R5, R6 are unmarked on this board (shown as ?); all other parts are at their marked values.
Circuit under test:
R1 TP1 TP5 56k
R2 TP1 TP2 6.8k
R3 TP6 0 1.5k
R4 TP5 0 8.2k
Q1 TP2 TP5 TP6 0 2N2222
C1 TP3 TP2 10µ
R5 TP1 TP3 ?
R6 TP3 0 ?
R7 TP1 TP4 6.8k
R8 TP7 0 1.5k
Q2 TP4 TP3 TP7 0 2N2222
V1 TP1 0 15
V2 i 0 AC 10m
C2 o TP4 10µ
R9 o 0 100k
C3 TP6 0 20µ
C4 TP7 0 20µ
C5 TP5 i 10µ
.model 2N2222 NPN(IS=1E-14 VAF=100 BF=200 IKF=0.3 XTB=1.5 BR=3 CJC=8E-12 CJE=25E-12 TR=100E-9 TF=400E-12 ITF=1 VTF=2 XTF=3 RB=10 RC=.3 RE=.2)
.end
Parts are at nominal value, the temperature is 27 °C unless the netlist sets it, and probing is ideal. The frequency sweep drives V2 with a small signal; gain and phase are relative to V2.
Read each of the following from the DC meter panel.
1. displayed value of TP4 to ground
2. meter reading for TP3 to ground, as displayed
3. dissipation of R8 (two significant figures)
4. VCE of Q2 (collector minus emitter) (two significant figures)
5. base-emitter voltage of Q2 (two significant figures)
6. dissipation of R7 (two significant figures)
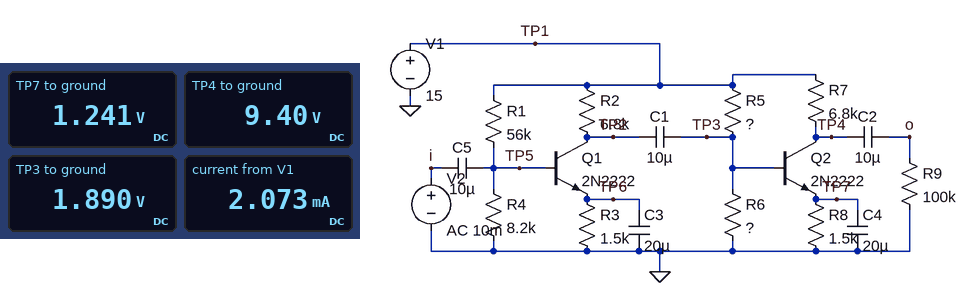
9.40 V
1.890 V
1.0 mW
8.2 V
650 mV
4.6 mW
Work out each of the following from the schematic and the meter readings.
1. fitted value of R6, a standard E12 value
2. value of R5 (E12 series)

10 kΩ
68 kΩ
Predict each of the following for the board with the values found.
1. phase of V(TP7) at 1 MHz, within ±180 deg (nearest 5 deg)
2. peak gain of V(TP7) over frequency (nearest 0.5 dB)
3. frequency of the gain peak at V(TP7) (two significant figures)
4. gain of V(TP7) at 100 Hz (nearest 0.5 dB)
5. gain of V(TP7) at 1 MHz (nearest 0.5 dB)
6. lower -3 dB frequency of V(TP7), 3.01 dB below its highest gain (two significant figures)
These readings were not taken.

15 deg
33.0 dB
200 Hz
31.0 dB
-56.0 dB
82 Hz
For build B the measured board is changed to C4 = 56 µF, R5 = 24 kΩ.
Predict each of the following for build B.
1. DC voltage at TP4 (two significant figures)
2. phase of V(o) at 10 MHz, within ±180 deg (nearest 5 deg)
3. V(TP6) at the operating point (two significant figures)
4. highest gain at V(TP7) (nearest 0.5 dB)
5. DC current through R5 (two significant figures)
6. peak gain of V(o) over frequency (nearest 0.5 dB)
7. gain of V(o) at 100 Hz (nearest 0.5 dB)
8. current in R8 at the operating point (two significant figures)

2.9 V
-145 deg
1.2 V
-9.0 dB
480 µA
15.0 dB
6.0 dB
1.9 mA
